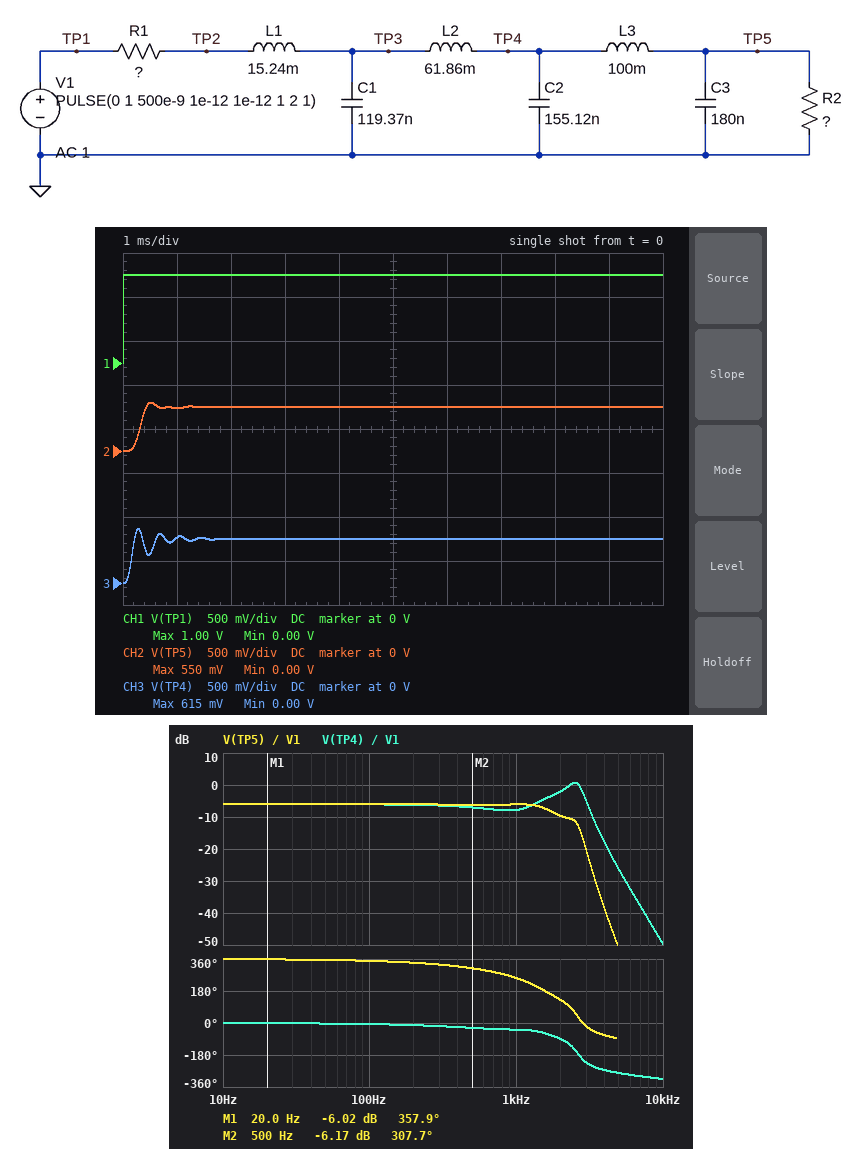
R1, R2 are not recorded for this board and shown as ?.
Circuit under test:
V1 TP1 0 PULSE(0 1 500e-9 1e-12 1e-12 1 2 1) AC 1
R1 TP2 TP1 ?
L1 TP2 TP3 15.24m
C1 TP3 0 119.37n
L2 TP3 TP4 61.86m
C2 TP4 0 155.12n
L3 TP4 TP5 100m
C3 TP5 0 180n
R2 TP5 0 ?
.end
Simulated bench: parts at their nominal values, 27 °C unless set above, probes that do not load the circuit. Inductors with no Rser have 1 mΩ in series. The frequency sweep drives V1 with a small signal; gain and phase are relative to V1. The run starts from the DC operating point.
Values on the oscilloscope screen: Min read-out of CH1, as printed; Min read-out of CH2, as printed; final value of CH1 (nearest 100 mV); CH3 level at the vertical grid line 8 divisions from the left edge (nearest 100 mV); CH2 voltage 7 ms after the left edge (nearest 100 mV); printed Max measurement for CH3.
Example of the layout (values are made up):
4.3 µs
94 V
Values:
0.00 V
0.00 V
1.0 V
500 mV
500 mV
615 mV
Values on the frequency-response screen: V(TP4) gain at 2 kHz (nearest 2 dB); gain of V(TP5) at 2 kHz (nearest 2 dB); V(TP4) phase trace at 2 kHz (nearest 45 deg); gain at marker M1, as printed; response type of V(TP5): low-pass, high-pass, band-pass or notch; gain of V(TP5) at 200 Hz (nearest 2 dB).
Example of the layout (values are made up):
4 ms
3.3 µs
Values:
-2 dB
-10 dB
-90 deg
-6.02 dB
low-pass
-6 dB
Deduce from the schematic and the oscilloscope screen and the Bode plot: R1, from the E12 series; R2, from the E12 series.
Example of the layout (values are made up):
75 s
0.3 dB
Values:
820 Ω
820 Ω
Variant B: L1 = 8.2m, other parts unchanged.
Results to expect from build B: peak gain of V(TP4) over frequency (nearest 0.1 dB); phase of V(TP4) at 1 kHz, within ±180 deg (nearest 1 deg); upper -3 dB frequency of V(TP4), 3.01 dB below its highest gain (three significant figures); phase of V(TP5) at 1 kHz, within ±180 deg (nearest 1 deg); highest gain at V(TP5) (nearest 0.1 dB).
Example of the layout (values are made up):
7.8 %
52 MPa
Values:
1.1 dB
-36 deg
2.79 kHz
-105 deg
-6.0 dB
